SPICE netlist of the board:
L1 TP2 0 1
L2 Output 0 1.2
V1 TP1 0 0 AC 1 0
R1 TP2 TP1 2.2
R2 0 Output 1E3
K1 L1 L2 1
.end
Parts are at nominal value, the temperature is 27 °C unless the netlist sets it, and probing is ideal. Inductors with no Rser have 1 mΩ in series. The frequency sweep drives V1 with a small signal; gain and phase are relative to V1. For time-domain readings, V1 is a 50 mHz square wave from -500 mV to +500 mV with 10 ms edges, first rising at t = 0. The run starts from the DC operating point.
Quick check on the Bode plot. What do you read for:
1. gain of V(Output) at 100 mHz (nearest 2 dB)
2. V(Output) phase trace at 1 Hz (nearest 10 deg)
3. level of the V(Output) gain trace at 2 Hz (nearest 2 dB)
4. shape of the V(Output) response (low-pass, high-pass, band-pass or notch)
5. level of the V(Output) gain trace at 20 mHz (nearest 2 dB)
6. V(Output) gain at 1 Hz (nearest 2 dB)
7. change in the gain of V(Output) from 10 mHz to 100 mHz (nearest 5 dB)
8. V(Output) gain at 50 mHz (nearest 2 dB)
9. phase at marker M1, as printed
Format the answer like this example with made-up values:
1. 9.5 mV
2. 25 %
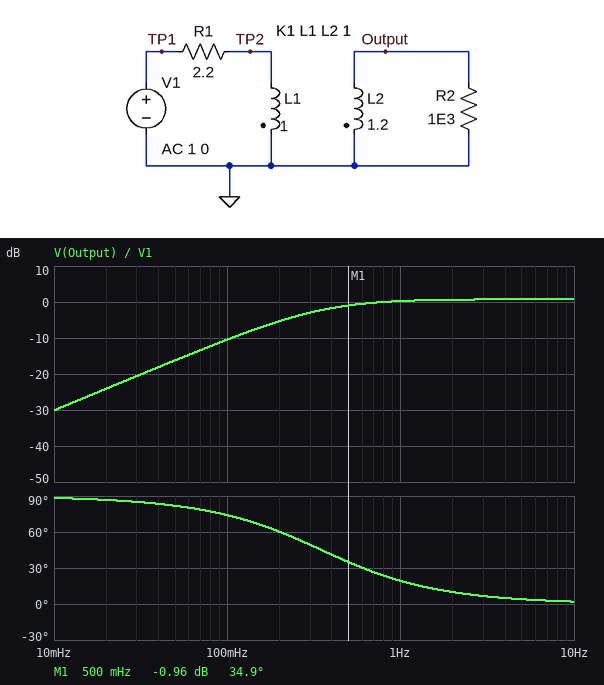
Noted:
1. -10 dB
2. 20 deg
3. 0 dB
4. high-pass
5. -24 dB
6. 0 dB
7. 20 dB
8. -16 dB
9. 34.9 deg
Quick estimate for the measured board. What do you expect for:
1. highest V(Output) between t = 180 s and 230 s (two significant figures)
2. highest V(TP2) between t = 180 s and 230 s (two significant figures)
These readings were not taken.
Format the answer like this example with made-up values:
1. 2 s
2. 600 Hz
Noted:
1. 1.1 V
2. 990 mV
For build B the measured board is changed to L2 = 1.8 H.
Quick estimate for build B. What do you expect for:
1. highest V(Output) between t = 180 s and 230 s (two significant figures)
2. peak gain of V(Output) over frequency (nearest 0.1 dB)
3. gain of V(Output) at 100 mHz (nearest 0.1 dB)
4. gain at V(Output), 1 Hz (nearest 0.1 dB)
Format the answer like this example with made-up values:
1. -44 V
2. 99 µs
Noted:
1. 1.3 V
2. 2.5 dB
3. -8.7 dB
4. 2.0 dB
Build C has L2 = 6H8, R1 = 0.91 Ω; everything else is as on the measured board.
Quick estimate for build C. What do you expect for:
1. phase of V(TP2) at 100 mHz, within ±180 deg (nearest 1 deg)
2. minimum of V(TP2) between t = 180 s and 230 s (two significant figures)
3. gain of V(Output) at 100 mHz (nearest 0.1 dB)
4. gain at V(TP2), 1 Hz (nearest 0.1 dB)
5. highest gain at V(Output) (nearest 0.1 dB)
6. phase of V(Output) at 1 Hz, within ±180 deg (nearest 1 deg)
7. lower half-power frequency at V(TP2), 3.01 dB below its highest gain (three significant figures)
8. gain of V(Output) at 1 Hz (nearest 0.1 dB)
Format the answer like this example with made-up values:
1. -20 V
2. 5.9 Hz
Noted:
1. 55 deg
2. -990 mV
3. 3.4 dB
4. -0.1 dB
5. 8.3 dB
6. 8 deg
7. 144 mHz
8. 8.2 dB
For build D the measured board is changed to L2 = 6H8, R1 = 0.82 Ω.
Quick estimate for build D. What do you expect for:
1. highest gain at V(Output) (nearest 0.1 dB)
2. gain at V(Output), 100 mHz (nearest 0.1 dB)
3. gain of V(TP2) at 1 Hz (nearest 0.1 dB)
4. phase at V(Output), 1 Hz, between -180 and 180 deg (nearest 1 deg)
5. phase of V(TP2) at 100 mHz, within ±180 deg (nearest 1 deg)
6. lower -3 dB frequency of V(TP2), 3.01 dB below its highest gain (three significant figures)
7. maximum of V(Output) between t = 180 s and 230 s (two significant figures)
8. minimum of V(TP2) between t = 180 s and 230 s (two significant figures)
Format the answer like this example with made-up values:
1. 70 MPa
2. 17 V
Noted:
1. 8.3 dB
2. 4.0 dB
3. -0.1 dB
4. 7 deg
5. 52 deg
6. 130 mHz
7. 2.6 V
8. -990 mV
